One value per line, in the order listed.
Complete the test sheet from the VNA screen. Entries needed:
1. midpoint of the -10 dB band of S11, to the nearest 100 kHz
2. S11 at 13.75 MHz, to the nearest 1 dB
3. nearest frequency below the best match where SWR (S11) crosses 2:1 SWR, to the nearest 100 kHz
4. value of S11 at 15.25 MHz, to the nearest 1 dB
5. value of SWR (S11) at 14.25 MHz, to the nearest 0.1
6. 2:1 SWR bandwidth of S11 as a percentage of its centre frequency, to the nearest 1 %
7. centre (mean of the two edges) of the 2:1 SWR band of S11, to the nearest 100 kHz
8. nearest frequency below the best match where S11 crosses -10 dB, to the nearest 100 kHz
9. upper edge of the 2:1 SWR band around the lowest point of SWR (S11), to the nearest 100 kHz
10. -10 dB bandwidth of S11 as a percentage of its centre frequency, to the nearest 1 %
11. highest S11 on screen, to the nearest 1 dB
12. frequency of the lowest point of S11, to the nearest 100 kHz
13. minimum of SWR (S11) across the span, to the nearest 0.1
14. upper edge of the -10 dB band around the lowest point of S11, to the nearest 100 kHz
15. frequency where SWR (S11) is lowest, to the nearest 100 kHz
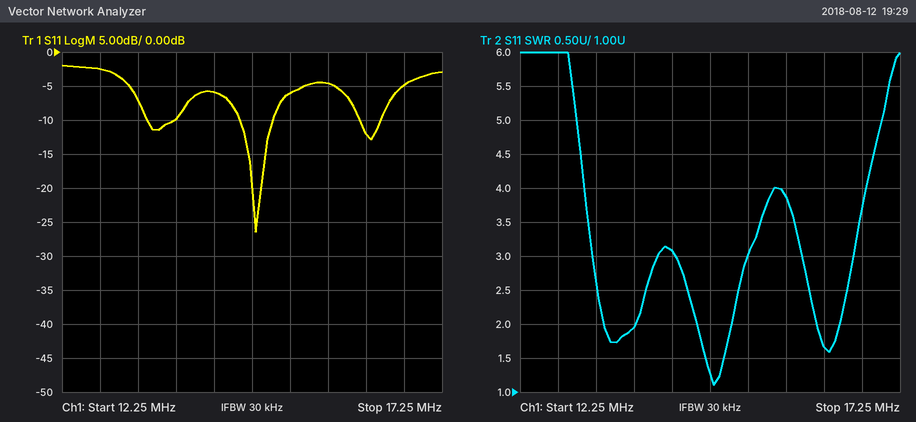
14.8 MHz
-10 dB
14.6 MHz
-6 dB
3.1
3 %
14.8 MHz
14.6 MHz
15.0 MHz
3 %
-2 dB
14.8 MHz
1.1
15.0 MHz
14.8 MHz
